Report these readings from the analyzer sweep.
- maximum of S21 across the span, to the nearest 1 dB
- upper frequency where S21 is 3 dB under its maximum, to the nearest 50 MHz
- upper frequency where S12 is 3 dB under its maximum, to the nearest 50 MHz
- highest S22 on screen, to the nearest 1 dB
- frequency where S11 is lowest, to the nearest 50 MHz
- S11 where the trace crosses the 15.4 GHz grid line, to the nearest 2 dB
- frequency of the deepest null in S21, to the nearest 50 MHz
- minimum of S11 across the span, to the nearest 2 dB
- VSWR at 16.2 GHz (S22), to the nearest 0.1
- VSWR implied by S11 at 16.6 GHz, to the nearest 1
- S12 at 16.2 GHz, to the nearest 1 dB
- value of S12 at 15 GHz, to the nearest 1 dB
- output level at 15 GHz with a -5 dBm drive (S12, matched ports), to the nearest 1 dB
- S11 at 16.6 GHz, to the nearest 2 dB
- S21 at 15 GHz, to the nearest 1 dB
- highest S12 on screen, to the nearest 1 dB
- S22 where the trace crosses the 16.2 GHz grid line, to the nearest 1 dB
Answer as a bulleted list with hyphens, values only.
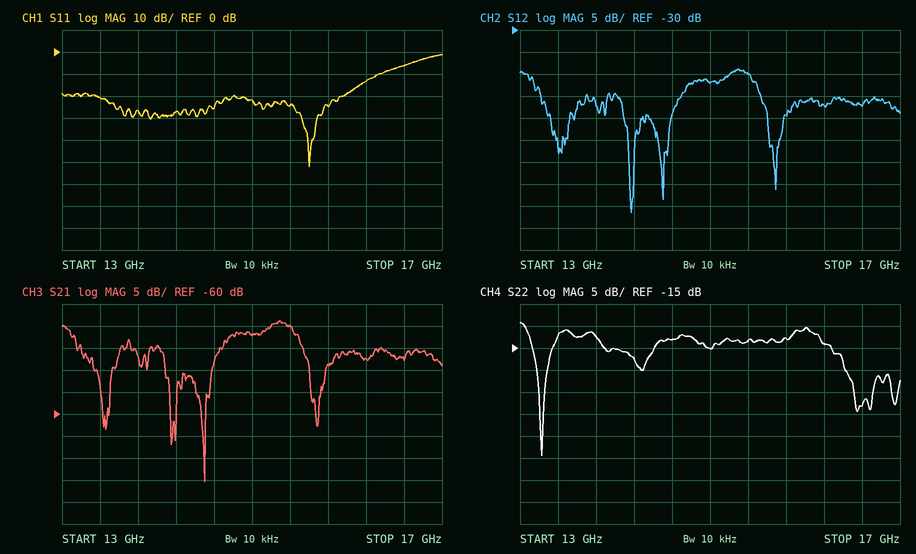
- -39 dB
- 15.45 GHz
- 15.50 GHz
- -9 dB
- 15.60 GHz
- -24 dB
- 14.50 GHz
- -52 dB
- 1.5
- 3
- -47 dB
- -42 dB
- -47 dBm
- -6 dB
- -42 dB
- -39 dB
- -14 dB
